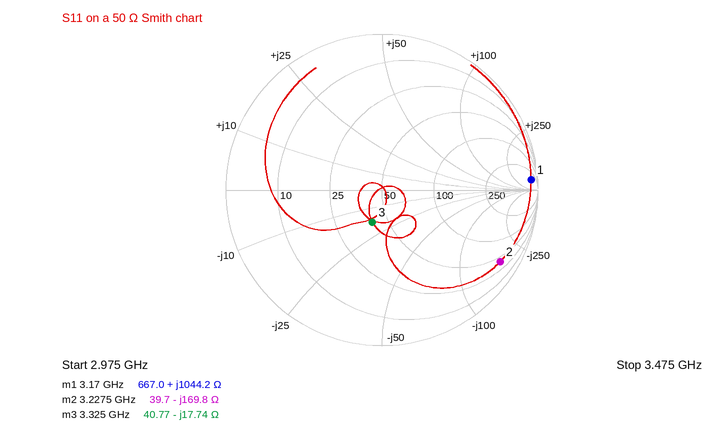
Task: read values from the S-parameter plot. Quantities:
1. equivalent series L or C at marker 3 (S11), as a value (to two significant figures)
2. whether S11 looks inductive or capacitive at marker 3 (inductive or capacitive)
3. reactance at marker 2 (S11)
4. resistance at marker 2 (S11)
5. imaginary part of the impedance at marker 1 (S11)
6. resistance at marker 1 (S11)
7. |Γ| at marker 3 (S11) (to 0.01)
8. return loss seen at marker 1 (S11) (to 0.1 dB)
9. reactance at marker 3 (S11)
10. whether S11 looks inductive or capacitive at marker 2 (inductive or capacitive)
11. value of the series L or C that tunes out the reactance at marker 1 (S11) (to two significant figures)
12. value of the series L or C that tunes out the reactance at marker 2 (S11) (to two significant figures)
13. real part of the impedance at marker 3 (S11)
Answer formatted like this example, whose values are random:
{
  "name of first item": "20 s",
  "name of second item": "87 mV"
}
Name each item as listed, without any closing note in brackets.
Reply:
{
  "equivalent series L or C at marker 3 (S11), as a value": "2.7 pF",
  "whether S11 looks inductive or capacitive at marker 3": "capacitive",
  "reactance at marker 2": "-169.8 Ω",
  "resistance at marker 2": "39.7 Ω",
  "imaginary part of the impedance at marker 1": "+1044.2 Ω",
  "resistance at marker 1": "667.0 Ω",
  "|Γ| at marker 3 (S11)": "0.22",
  "return loss seen at marker 1 (S11)": "0.4 dB",
  "reactance at marker 3": "-17.74 Ω",
  "whether S11 looks inductive or capacitive at marker 2": "capacitive",
  "value of the series L or C that tunes out the reactance at marker 1 (S11)": "48 fF",
  "value of the series L or C that tunes out the reactance at marker 2 (S11)": "8.4 nH",
  "real part of the impedance at marker 3": "40.77 Ω"
}
